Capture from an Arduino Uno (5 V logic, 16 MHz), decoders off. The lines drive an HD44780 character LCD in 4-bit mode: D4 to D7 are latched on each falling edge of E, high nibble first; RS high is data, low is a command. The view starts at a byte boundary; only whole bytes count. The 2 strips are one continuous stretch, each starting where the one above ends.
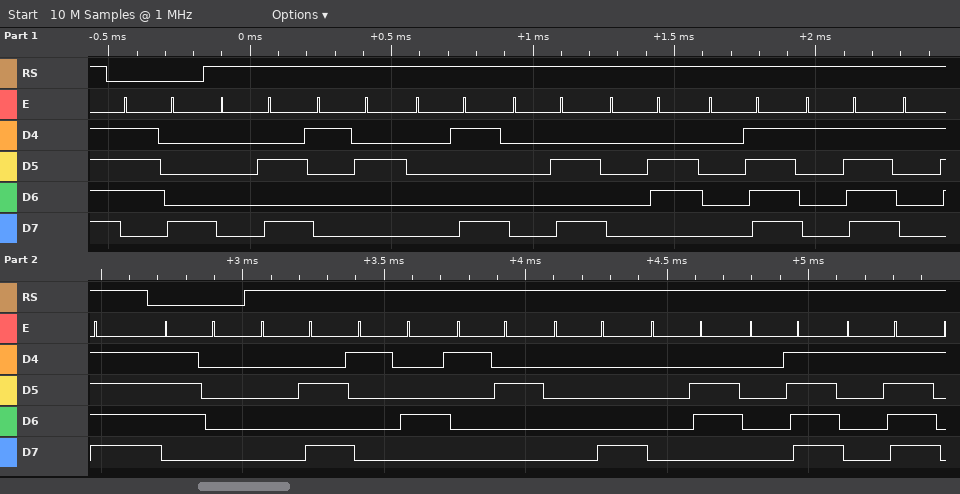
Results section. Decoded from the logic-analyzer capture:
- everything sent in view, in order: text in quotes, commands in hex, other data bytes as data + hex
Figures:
0x78 data 0A 12 09 0A 06 0F 1F 1F 0x70 data 0A 14 12 08 06 0F 1F
